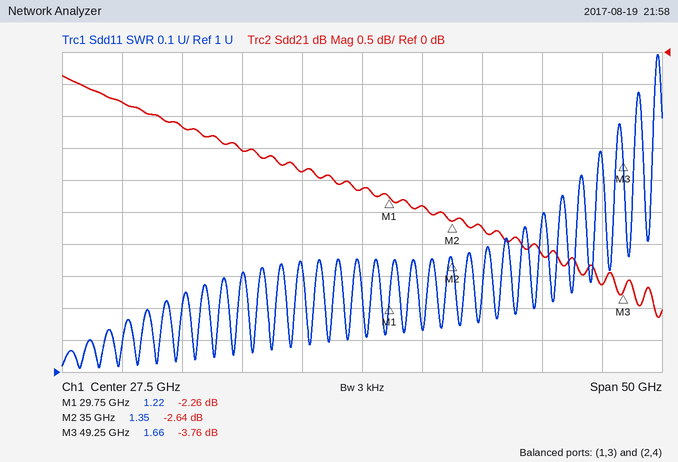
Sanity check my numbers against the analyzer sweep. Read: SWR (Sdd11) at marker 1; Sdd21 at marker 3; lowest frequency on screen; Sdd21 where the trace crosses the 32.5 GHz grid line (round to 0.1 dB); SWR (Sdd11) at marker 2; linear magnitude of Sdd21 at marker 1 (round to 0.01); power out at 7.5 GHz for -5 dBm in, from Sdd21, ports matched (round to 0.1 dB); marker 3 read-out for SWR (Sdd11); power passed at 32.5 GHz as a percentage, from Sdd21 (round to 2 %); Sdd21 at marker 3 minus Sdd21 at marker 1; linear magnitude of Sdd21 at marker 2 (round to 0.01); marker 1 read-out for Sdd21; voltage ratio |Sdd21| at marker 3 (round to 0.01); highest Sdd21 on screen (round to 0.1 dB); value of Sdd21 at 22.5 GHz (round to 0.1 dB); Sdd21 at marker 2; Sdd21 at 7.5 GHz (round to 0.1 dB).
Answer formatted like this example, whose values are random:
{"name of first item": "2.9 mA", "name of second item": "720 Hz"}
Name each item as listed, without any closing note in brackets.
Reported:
{"SWR (Sdd11) at marker 1": "1.22", "Sdd21 at marker 3": "-3.76 dB", "lowest frequency on screen": "2.5 GHz", "Sdd21 where the trace crosses the 32.5 GHz grid line": "-2.4 dB", "SWR (Sdd11) at marker 2": "1.35", "linear magnitude of Sdd21 at marker 1": "0.77", "power out at 7.5 GHz for -5 dBm in, from Sdd21, ports matched": "-5.8 dBm", "marker 3 read-out for SWR": "1.66", "power passed at 32.5 GHz as a percentage, from Sdd21": "58 %", "Sdd21 at marker 3 minus Sdd21 at marker 1": "-1.50 dB", "linear magnitude of Sdd21 at marker 2": "0.74", "marker 1 read-out for Sdd21": "-2.26 dB", "voltage ratio |Sdd21| at marker 3": "0.65", "highest Sdd21 on screen": "-0.4 dB", "value of Sdd21 at 22.5 GHz": "-1.9 dB", "Sdd21 at marker 2": "-2.64 dB", "Sdd21 at 7.5 GHz": "-0.8 dB"}
